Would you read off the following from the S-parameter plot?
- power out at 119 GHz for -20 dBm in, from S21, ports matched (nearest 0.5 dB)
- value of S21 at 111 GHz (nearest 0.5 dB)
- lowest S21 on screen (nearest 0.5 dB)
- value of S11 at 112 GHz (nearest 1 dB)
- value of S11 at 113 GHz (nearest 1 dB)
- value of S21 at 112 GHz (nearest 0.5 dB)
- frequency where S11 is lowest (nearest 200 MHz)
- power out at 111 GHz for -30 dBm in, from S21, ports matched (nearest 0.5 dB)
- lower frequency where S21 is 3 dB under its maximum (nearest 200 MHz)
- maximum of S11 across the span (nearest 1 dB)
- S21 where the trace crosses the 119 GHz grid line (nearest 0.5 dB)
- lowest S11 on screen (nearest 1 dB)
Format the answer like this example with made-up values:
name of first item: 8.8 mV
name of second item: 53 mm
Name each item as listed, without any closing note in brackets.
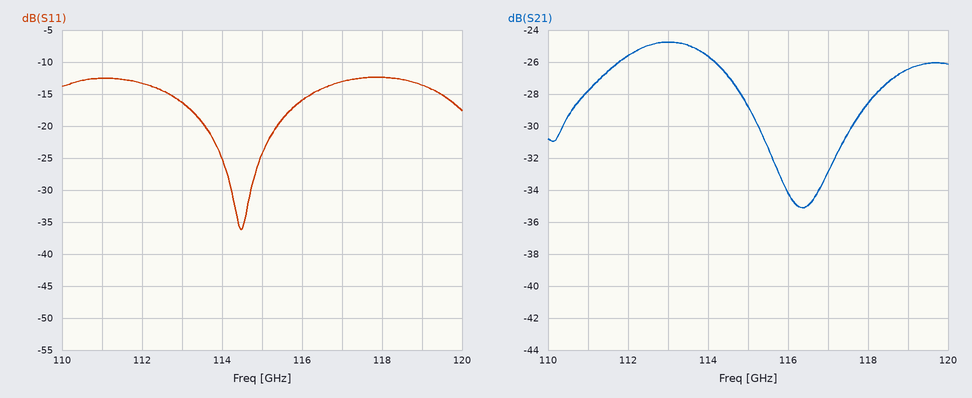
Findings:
power out at 119 GHz for -20 dBm in, from S21, ports matched: -46.5 dBm
value of S21 at 111 GHz: -28.0 dB
lowest S21 on screen: -35.0 dB
value of S11 at 112 GHz: -13 dB
value of S11 at 113 GHz: -16 dB
value of S21 at 112 GHz: -25.5 dB
frequency where S11 is lowest: 114.4 GHz
power out at 111 GHz for -30 dBm in, from S21, ports matched: -58.0 dBm
lower frequency where S21 is 3 dB under its maximum: 111.0 GHz
maximum of S11 across the span: -12 dB
S21 where the trace crosses the 119 GHz grid line: -26.5 dB
lowest S11 on screen: -36 dB
